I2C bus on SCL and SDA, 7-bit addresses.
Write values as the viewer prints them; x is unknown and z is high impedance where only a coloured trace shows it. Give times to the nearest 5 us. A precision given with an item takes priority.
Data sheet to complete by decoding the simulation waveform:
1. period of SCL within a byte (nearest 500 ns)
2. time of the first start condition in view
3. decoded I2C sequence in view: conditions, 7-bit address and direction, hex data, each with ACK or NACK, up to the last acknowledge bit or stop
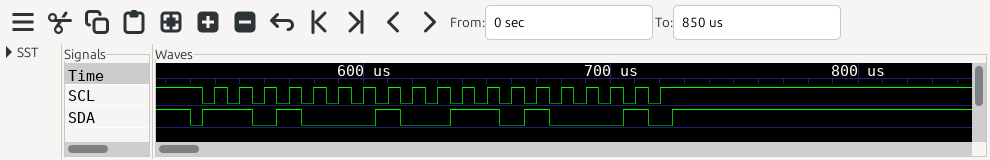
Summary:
10000 ns
530 us
start, address 68 read ACK, 68 NACK, stop
